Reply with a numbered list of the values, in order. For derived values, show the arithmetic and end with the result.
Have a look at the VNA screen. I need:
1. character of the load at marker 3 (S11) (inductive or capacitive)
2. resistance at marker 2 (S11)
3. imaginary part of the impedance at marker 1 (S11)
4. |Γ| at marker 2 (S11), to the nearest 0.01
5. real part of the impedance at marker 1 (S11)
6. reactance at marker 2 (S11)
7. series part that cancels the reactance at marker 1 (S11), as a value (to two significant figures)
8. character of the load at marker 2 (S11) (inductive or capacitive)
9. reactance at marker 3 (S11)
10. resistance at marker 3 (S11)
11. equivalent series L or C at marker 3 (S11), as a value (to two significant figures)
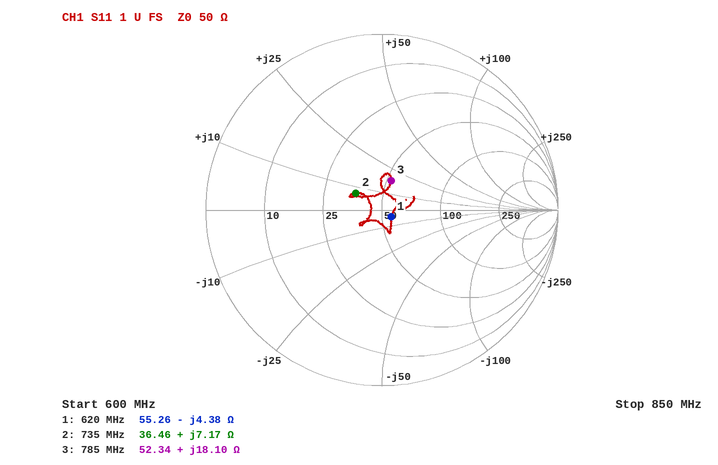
1. inductive
2. 36.46 Ω
3. -4.38 Ω
4. 0.18
5. 55.26 Ω
6. +7.17 Ω
7. L = 4.38 Ω/(2π × 620 MHz) ≈ 1.1 nH
8. inductive
9. +18.10 Ω
10. 52.34 Ω
11. L = 18.1 Ω/(2π × 785 MHz) ≈ 3.7 nH
